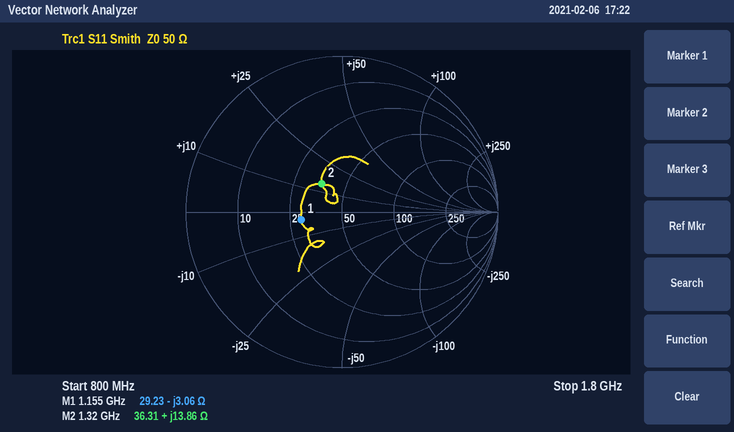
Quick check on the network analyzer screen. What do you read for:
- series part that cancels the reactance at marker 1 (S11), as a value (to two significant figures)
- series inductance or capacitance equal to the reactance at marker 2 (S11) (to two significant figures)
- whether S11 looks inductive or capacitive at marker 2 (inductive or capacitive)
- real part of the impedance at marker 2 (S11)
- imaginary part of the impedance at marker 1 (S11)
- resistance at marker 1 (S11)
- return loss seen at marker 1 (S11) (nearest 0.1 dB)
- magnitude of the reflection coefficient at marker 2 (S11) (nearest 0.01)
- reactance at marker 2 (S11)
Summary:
420 pH
1.7 nH
inductive
36.31 Ω
-3.06 Ω
29.23 Ω
11.5 dB
0.22
+13.86 Ω
